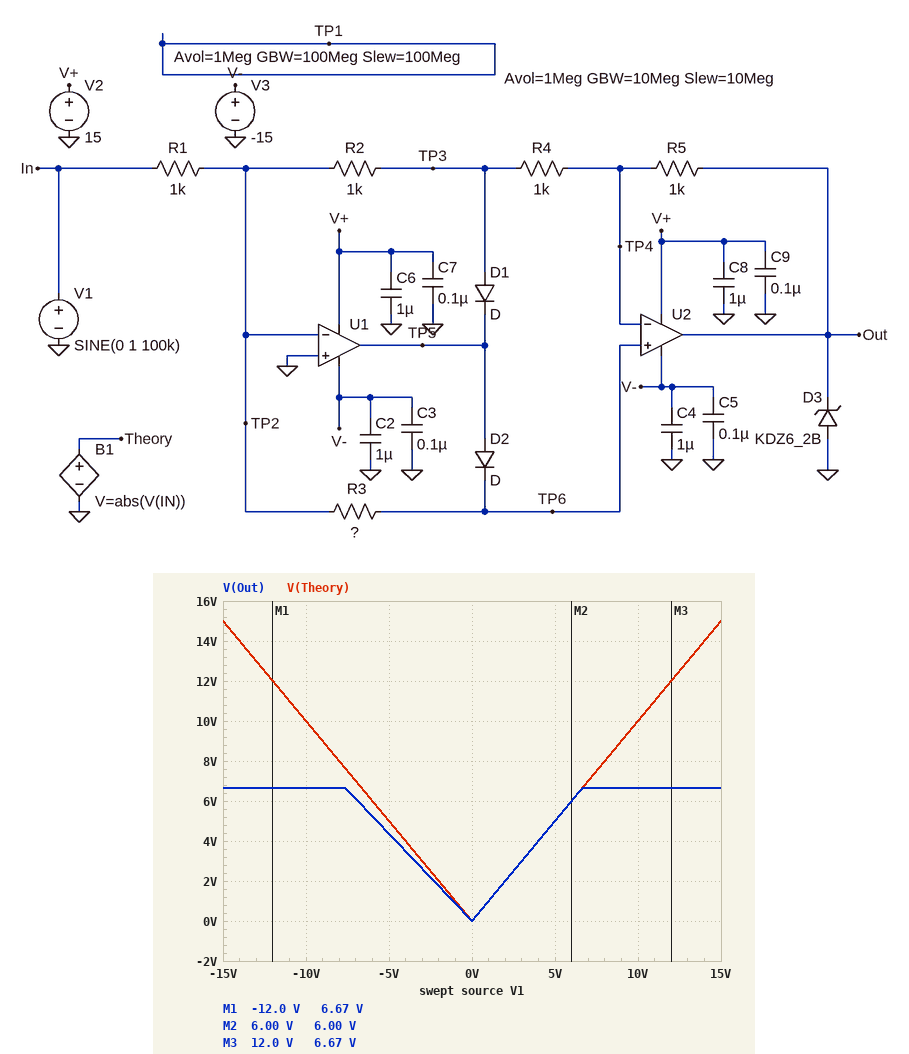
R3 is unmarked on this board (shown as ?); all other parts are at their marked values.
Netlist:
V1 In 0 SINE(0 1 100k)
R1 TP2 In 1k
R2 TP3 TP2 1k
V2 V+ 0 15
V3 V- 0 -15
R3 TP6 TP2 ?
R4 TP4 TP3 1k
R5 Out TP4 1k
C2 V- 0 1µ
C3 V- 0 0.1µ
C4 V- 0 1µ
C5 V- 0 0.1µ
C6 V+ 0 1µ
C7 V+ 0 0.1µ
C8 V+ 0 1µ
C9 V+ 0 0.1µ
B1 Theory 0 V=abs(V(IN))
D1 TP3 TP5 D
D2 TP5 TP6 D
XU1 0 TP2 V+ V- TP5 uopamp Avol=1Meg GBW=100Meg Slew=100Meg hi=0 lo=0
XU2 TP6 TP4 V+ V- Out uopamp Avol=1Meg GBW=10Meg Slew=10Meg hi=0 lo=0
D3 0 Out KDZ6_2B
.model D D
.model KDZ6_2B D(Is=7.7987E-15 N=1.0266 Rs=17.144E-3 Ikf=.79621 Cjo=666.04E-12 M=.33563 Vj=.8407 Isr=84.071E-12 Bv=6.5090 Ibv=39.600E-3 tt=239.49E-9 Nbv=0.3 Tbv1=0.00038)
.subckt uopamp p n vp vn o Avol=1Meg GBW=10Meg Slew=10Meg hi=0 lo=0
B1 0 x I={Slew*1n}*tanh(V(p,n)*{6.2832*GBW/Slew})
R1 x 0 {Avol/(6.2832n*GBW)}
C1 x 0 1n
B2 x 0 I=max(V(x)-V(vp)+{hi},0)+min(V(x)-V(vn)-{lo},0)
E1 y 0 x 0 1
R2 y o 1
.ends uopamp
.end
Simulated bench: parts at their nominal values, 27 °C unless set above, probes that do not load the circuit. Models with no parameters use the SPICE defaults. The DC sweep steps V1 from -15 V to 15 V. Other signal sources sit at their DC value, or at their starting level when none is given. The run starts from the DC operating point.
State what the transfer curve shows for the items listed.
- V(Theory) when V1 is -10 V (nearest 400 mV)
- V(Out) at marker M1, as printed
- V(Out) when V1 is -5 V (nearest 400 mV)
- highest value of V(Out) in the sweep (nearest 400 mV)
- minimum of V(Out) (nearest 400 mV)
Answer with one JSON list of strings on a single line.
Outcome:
["10.0 V", "6.67 V", "4.4 V", "6.8 V", "0 V"]
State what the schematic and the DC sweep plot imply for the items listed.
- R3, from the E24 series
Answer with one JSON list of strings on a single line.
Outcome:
["820 Ω"]
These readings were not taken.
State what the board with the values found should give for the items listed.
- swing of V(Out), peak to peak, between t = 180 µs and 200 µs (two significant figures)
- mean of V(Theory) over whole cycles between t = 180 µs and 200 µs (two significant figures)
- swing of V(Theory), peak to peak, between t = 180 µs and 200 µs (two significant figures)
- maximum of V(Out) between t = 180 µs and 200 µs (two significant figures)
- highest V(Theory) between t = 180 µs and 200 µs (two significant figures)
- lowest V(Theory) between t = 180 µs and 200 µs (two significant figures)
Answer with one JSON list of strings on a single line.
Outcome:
["1.0 V", "640 mV", "1.0 V", "1.0 V", "1.0 V", "1.3 mV"]
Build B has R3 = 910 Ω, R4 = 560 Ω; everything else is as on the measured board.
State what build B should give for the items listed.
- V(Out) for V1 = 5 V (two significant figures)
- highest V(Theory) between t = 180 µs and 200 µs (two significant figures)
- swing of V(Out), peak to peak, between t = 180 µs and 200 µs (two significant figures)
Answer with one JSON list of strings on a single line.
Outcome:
["6.7 V", "1.0 V", "1.8 V"]
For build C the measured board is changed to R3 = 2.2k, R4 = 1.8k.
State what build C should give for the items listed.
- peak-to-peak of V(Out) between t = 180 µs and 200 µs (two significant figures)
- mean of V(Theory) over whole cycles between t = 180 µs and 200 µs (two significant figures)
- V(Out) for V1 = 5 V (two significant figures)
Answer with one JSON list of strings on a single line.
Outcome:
["1.7 V", "640 mV", "2.8 V"]
